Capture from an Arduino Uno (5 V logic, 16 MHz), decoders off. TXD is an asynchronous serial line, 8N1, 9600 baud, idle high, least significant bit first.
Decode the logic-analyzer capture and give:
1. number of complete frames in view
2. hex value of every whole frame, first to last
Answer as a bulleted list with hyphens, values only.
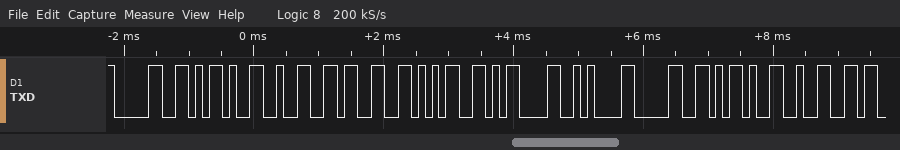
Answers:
- 10
- 0x30 0x2D 0x32 0x33 0x35 0x0D 0x0A 0x30 0x2D 0x32
